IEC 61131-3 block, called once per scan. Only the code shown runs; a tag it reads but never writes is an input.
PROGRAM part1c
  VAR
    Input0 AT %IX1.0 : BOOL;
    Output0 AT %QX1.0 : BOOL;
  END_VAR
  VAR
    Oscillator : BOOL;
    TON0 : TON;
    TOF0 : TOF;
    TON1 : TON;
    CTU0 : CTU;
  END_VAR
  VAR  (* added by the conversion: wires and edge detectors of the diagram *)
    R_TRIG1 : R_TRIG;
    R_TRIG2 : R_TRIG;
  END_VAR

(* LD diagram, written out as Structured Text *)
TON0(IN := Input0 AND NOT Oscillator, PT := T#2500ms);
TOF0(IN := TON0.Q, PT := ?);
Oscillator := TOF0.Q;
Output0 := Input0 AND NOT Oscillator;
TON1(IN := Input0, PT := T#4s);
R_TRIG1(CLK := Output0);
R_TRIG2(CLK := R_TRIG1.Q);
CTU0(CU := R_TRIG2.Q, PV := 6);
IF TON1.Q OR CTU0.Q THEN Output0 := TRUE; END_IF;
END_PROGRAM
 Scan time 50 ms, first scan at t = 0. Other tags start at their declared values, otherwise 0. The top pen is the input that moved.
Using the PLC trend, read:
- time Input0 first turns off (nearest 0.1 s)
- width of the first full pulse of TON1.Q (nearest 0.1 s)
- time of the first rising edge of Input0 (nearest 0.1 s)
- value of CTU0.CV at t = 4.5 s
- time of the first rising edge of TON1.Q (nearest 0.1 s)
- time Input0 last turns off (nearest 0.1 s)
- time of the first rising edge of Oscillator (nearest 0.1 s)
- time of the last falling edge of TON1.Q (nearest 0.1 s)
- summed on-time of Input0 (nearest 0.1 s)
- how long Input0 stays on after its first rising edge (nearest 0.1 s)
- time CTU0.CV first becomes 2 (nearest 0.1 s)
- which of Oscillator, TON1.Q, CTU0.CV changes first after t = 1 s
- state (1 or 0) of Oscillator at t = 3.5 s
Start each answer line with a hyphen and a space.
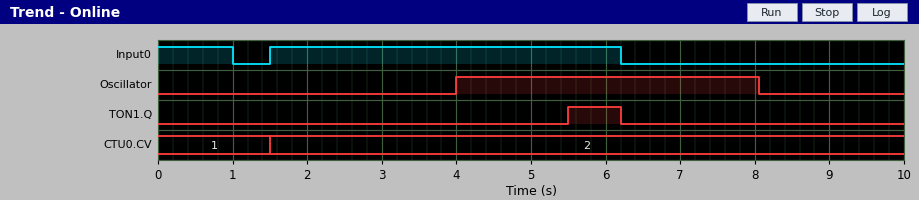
- 1.0 s
- 0.7 s
- 1.5 s
- 2
- 5.5 s
- 6.2 s
- 4.0 s
- 6.2 s
- 5.7 s
- 4.7 s
- 1.5 s
- CTU0.CV
- 0
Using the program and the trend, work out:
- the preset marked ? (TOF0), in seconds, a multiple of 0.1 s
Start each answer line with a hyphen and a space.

- 4.0 s
